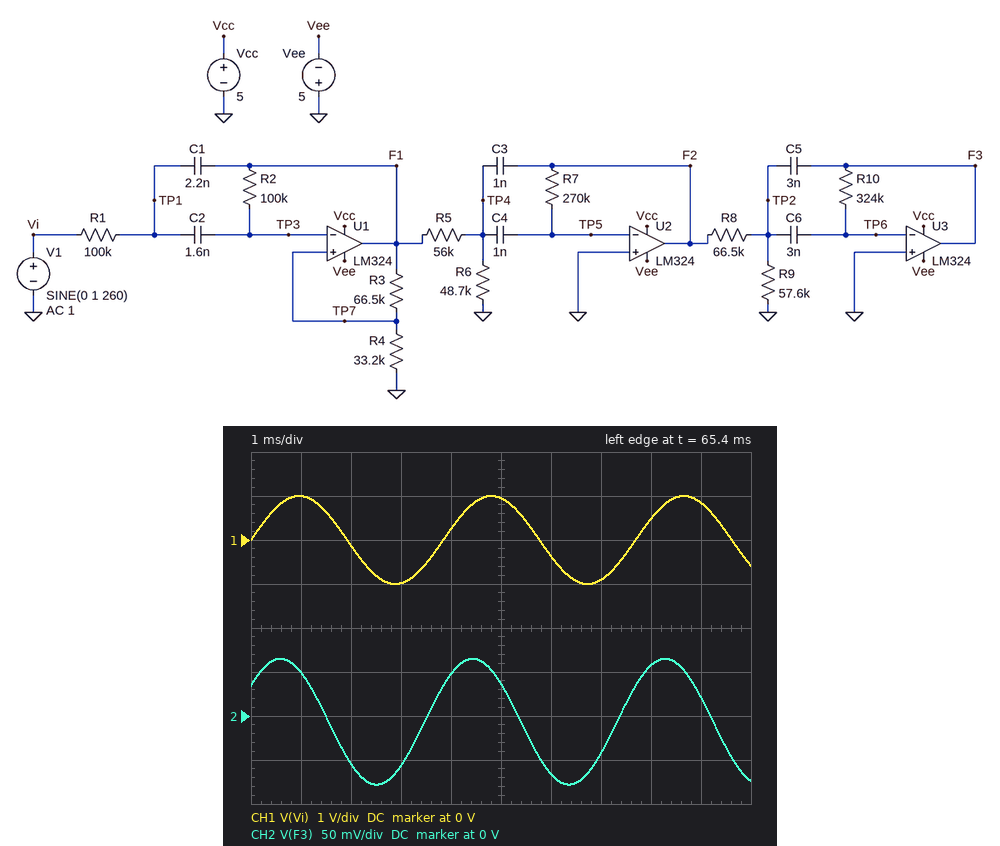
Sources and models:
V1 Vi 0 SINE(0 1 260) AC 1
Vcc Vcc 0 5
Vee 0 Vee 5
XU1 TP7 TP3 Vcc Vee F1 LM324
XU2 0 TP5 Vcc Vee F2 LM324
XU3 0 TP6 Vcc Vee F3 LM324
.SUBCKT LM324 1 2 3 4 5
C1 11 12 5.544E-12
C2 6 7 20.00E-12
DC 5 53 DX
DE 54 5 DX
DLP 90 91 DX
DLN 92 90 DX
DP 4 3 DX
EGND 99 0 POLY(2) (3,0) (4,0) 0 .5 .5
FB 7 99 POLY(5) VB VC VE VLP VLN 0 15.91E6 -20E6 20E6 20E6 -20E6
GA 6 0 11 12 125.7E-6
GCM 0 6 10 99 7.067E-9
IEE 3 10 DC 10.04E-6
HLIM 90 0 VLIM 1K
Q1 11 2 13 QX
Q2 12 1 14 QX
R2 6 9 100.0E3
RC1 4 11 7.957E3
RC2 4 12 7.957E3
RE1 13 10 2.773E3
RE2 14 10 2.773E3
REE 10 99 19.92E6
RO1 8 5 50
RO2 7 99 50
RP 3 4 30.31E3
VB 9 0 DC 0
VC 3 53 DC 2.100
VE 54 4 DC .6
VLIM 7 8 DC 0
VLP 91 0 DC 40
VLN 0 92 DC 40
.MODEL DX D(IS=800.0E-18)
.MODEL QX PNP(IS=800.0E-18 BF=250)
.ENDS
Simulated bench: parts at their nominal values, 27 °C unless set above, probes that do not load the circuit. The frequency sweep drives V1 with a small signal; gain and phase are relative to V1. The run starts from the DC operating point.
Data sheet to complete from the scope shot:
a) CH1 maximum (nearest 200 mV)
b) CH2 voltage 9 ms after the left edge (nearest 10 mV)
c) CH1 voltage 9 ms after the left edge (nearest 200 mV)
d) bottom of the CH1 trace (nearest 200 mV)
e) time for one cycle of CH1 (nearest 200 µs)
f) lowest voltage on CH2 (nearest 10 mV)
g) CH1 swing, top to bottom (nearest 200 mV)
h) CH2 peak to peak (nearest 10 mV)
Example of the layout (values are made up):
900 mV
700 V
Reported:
1.0 V
20 mV
800 mV
-1.0 V
3.8 ms
-80 mV
2.0 V
140 mV
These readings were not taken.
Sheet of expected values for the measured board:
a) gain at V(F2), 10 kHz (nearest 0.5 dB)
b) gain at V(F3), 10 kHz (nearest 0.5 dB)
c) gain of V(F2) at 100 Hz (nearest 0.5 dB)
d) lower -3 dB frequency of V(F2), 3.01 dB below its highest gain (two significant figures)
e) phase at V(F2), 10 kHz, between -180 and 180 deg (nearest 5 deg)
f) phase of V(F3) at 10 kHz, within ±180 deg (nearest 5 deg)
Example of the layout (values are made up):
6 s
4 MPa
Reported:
-30.0 dB
-52.0 dB
-38.5 dB
1.2 kHz
-165 deg
-75 deg
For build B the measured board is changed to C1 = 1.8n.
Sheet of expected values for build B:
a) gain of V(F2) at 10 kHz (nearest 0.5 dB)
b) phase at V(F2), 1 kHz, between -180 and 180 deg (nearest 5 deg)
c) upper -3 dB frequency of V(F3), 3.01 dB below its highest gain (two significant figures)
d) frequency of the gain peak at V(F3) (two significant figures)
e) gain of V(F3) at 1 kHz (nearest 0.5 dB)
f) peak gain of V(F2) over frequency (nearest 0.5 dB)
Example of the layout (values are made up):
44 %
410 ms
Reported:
-28.5 dB
60 deg
1.9 kHz
700 Hz
-0.5 dB
4.0 dB
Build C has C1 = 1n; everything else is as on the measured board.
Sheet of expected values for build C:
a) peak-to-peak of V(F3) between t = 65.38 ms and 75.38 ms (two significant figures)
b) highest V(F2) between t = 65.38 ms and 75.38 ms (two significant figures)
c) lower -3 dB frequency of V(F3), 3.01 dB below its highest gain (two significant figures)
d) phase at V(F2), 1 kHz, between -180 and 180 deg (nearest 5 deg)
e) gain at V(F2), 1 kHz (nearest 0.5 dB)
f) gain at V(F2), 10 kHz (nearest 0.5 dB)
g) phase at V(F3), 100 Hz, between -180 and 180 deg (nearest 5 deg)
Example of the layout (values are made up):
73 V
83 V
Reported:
150 mV
76 mV
610 Hz
85 deg
2.0 dB
-23.0 dB
75 deg
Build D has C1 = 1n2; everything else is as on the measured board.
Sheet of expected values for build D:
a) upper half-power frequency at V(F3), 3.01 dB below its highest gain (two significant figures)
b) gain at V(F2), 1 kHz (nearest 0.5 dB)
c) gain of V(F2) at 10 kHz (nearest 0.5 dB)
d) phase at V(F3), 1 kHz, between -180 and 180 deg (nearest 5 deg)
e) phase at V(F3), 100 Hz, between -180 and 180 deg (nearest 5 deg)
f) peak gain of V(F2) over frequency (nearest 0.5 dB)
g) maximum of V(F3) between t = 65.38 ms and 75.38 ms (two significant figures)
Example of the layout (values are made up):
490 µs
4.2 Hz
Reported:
2.0 kHz
1.5 dB
-25.0 dB
-170 deg
75 deg
7.5 dB
67 mV
